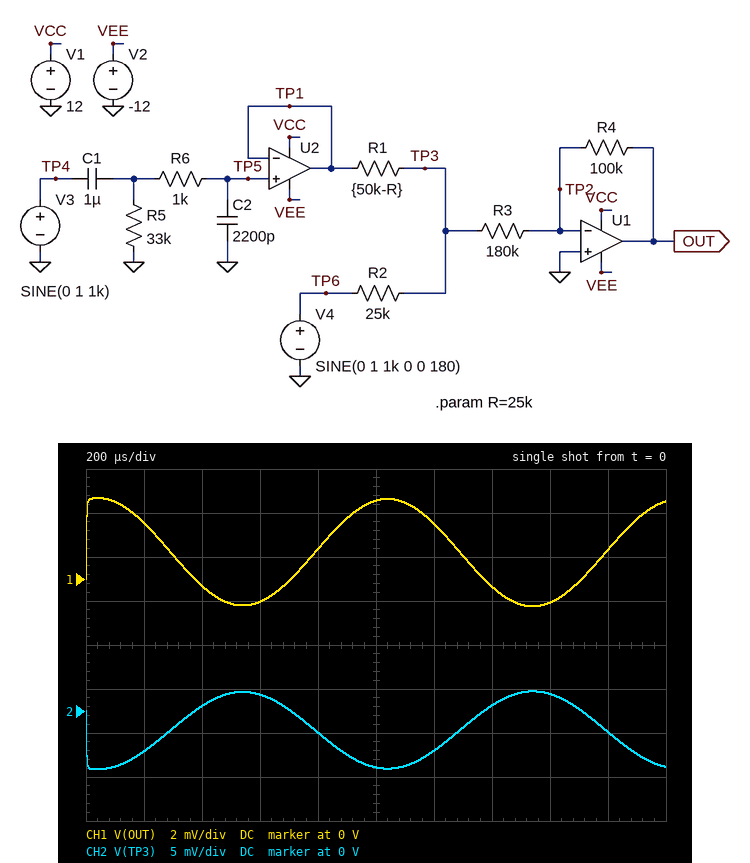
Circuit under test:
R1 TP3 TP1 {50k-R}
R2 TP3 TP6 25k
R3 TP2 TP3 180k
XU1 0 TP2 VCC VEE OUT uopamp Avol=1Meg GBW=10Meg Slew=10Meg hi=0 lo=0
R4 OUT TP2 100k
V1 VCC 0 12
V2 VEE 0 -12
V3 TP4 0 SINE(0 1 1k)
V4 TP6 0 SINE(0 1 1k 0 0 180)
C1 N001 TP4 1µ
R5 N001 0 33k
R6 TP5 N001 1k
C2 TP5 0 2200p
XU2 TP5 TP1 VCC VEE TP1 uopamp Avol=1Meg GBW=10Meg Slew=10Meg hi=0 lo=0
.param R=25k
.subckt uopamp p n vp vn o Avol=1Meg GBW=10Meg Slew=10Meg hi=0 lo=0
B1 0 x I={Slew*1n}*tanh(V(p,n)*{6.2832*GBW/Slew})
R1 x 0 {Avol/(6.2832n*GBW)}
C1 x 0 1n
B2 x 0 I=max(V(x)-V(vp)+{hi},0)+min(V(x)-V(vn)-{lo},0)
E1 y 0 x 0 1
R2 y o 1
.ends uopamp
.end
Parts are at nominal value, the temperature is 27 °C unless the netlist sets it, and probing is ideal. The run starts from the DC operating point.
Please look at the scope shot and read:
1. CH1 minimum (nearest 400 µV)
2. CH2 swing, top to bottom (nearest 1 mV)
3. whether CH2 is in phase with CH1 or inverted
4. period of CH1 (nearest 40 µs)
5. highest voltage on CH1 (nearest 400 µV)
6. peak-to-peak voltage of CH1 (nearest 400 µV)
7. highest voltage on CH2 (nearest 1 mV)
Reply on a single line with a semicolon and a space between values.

-1.2 mV; 9 mV; inverted; 1.00 ms; 3.6 mV; 4.8 mV; 2 mV
